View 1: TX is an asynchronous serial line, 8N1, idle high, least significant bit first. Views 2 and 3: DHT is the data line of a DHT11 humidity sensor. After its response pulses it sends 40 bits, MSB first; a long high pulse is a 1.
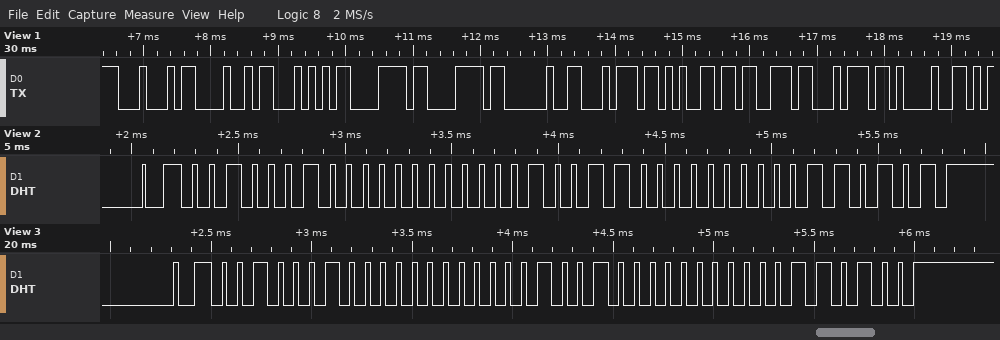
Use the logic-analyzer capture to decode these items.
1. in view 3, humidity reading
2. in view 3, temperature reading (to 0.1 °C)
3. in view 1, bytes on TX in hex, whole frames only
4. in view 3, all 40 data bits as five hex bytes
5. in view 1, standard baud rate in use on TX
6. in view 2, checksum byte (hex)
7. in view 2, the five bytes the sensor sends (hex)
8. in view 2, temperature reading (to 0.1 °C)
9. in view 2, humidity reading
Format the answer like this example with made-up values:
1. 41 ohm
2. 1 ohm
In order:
1. 34 %
2. 18.0 °C
3. 44 48 54 78 78 20 74 65 73 74 21
4. 22 00 12 00 34
5. 9600 baud
6. 0x35
7. 22 00 13 00 35
8. 19.0 °C
9. 34 %
